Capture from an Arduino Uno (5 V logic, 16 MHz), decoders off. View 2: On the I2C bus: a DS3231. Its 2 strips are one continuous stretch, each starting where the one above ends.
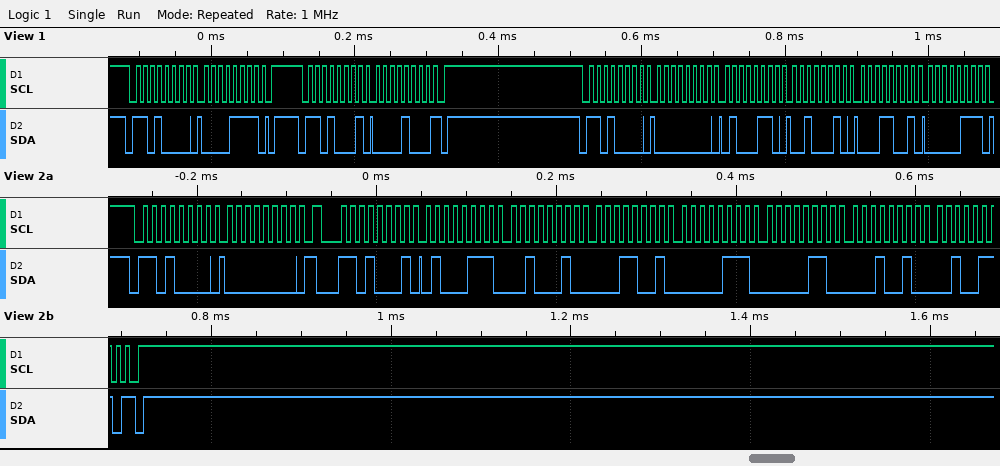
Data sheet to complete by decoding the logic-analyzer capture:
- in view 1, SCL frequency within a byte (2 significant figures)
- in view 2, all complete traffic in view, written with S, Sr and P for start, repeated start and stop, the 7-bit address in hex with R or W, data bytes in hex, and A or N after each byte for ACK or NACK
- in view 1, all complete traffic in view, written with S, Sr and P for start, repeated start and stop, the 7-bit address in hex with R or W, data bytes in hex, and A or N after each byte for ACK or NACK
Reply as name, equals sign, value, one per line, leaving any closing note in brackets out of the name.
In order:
in view 1, SCL frequency within a byte = 100 kHz
in view 2, all complete traffic in view, written with S, Sr and P for start, repeated start and stop, the 7-bit address in hex with R or W, data bytes in hex, and A or N after each byte for ACK or NACK = S 68W A 00 A Sr 68R A 47 A 22 A 19 A 07 A 06 A 12 A 26 N P
in view 1, all complete traffic in view, written with S, Sr and P for start, repeated start and stop, the 7-bit address in hex with R or W, data bytes in hex, and A or N after each byte for ACK or NACK = S 68W A 0F A P S 68R A 08 N P S 68W A 00 A 46 A 22 A 19 A 07 A
